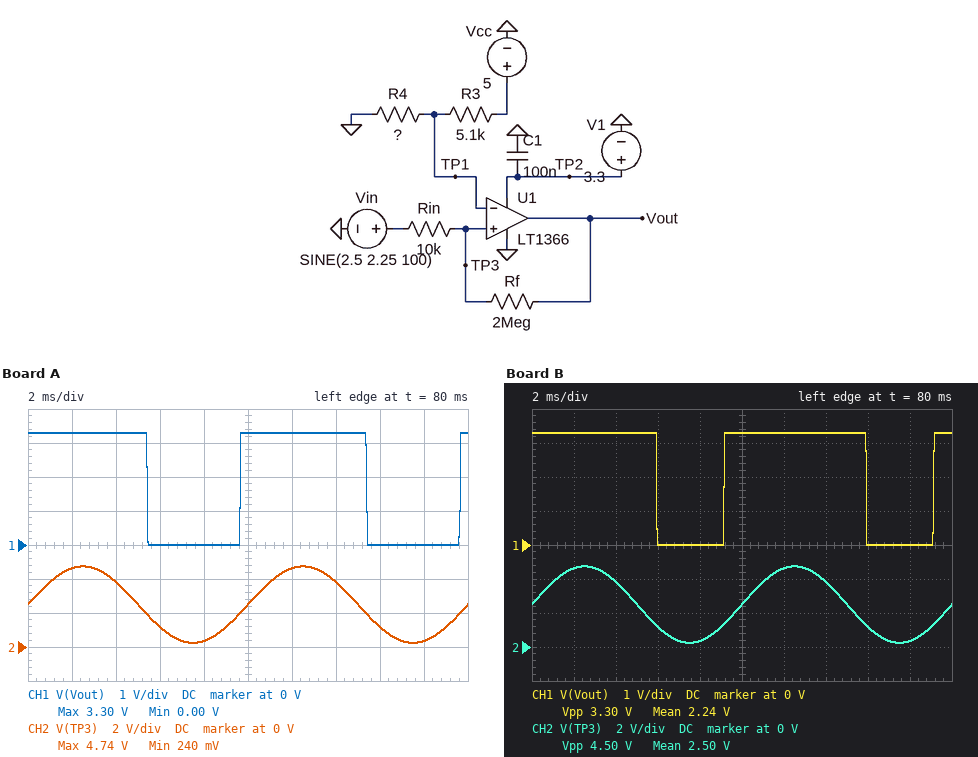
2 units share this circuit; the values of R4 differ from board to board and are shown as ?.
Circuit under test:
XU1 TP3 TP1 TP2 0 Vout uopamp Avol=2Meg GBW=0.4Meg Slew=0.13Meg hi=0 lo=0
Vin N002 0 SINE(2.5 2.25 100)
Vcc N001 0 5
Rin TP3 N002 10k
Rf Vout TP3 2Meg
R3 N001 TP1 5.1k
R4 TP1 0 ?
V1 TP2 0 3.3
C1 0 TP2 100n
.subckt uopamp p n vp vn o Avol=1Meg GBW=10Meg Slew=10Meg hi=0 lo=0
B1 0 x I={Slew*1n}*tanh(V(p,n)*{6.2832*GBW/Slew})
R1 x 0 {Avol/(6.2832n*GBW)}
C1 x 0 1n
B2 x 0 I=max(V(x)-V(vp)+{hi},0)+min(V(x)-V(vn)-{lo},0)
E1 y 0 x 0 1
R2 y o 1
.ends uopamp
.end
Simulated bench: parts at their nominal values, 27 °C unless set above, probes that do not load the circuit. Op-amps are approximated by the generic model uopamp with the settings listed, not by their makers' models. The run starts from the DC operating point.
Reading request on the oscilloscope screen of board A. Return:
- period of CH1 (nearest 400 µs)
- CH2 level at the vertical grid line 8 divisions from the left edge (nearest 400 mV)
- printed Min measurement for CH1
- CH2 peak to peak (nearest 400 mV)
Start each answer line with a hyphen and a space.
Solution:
- 10.0 ms
- 1.2 V
- 0.00 V
- 4.4 V
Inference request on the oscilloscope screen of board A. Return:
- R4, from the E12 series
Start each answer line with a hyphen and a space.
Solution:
- 3.3 kΩ
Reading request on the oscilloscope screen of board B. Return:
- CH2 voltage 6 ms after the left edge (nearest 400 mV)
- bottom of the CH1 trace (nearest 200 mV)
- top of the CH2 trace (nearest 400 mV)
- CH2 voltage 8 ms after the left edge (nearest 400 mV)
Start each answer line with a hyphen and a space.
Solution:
- 1.2 V
- 0 V
- 4.8 V
- 400 mV
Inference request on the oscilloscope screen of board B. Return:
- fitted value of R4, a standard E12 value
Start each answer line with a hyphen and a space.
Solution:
- 1.8 kΩ
